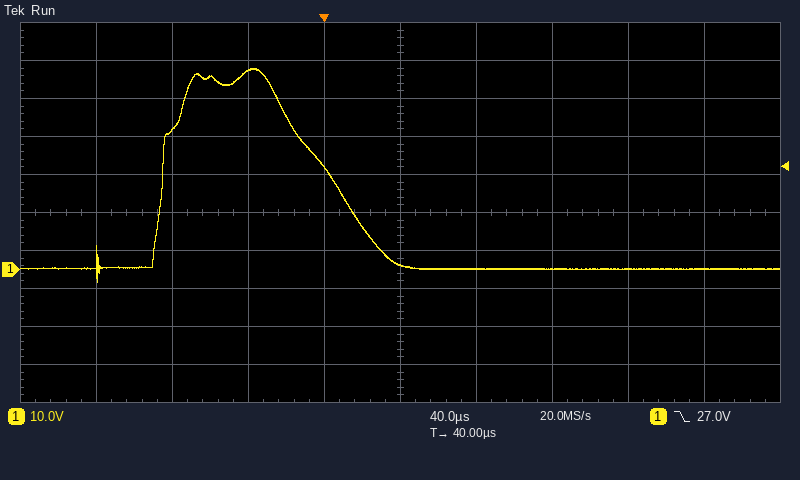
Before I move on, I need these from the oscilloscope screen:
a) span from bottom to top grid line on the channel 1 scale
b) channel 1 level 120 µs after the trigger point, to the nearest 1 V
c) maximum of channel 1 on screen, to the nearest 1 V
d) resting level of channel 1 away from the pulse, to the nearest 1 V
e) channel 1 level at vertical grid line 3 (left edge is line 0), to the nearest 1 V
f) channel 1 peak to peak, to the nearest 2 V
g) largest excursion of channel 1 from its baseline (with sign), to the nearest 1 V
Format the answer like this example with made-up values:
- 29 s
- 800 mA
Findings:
- 100 V
- 0 V
- 53 V
- 0 V
- 52 V
- 56 V
- +53 V
